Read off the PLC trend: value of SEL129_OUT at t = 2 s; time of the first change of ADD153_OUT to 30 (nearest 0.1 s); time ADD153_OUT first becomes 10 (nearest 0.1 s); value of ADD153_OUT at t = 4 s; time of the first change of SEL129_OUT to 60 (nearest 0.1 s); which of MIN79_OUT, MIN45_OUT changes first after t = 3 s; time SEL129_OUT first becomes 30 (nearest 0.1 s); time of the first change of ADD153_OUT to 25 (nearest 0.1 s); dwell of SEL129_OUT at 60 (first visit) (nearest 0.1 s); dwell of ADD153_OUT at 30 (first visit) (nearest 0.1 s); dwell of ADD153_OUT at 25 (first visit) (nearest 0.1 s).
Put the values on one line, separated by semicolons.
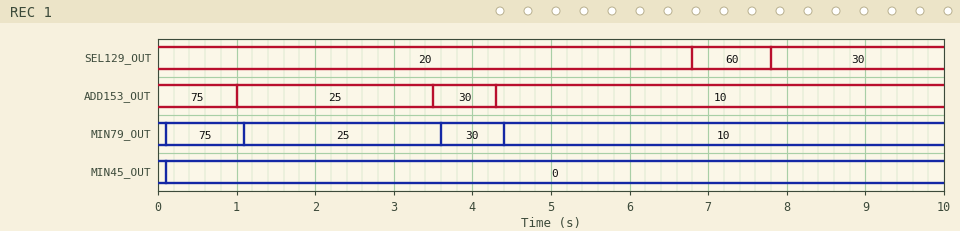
20; 3.5 s; 4.3 s; 30; 6.8 s; MIN79_OUT; 7.8 s; 1.0 s; 1.0 s; 0.8 s; 2.5 s
